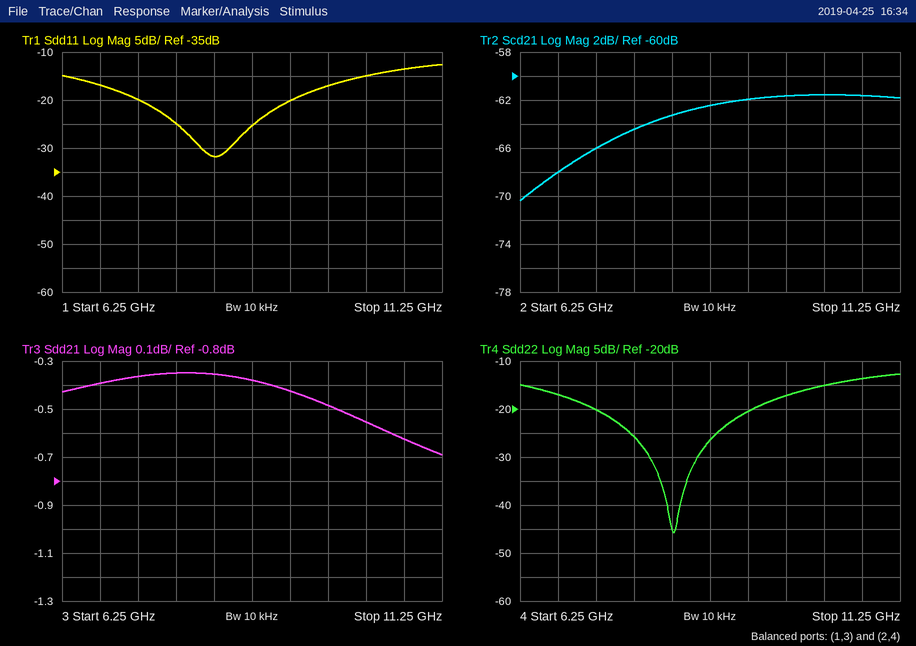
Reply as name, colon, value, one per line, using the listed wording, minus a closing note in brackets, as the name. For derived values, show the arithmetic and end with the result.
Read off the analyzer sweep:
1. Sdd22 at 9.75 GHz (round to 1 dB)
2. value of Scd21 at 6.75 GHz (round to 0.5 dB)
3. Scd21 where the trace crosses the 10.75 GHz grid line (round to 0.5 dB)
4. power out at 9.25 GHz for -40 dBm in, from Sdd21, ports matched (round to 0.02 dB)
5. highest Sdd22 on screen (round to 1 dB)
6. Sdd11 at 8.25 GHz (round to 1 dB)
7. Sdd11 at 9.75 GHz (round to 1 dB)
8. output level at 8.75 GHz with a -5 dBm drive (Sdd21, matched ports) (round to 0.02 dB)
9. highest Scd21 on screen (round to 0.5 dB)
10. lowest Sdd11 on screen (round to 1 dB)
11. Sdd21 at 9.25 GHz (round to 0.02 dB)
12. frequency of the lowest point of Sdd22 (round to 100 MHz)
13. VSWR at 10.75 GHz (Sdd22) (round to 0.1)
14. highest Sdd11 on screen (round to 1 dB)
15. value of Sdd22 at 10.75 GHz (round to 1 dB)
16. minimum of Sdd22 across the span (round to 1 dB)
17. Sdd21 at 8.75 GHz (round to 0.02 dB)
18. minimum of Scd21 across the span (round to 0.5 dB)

Sdd22 at 9.75 GHz: -17 dB
value of Scd21 at 6.75 GHz: -68.0 dB
Scd21 where the trace crosses the 10.75 GHz grid line: -61.5 dB
power out at 9.25 GHz for -40 dBm in, from Sdd21, ports matched: -40 dBm + (-0.42 dB) = -40.42 dBm
highest Sdd22 on screen: -13 dB
Sdd11 at 8.25 GHz: -32 dB
Sdd11 at 9.75 GHz: -17 dB
output level at 8.75 GHz with a -5 dBm drive (Sdd21, matched ports): -5 dBm + (-0.38 dB) = -5.38 dBm
highest Scd21 on screen: -61.5 dB
lowest Sdd11 on screen: -32 dB
Sdd21 at 9.25 GHz: -0.42 dB
frequency of the lowest point of Sdd22: 8.3 GHz
VSWR at 10.75 GHz (Sdd22): |Γ| = 10^(-14/20) = 0.1995; VSWR = (1 + 0.1995)/(1 − 0.1995) ≈ 1.5
highest Sdd11 on screen: -13 dB
value of Sdd22 at 10.75 GHz: -14 dB
minimum of Sdd22 across the span: -46 dB
Sdd21 at 8.75 GHz: -0.38 dB
minimum of Scd21 across the span: -70.5 dB
